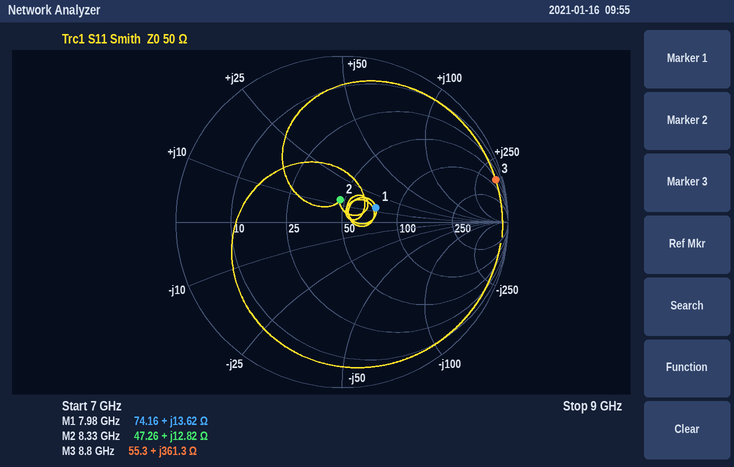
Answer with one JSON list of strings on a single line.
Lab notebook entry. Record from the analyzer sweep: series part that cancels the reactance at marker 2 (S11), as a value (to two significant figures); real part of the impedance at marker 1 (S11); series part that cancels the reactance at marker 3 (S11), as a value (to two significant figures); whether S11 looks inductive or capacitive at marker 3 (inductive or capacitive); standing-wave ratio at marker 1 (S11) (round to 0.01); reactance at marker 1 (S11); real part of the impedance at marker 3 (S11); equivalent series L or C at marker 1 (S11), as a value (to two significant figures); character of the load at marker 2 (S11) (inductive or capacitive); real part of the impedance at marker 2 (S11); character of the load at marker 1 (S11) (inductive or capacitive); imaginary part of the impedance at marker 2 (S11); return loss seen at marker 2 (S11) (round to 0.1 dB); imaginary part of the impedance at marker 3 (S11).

["1.5 pF", "74.16 Ω", "50 fF", "inductive", "1.57", "+13.62 Ω", "55.3 Ω", "270 pH", "inductive", "47.26 Ω", "inductive", "+12.82 Ω", "17.5 dB", "+361.3 Ω"]
